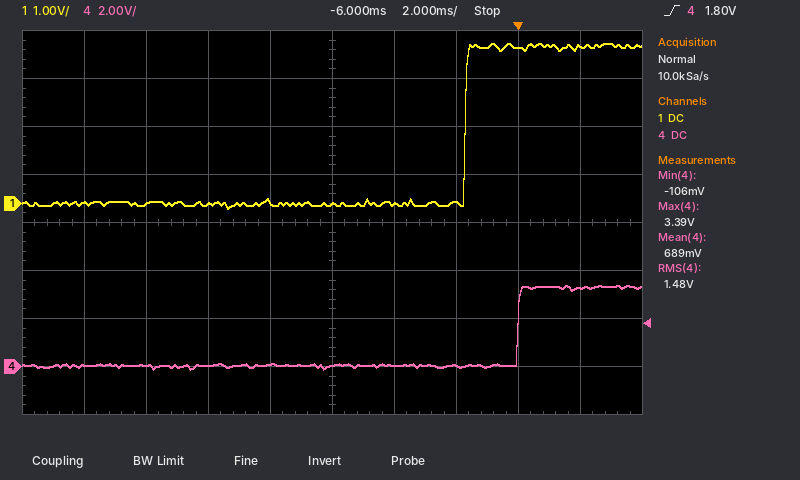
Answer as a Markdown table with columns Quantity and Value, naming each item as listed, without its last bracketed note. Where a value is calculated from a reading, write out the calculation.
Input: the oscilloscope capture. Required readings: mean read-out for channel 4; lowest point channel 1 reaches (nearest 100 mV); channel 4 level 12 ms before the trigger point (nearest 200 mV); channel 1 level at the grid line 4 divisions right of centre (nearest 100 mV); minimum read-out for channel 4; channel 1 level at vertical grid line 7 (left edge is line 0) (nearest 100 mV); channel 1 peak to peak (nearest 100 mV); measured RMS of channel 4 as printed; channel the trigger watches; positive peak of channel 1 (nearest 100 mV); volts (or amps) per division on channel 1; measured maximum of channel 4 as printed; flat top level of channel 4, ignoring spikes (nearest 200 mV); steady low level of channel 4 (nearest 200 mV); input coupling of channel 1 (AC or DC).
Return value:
| Quantity | Value |
|---|---|
| mean read-out for channel 4 | 689 mV |
| lowest point channel 1 reaches | -100 mV |
| channel 4 level 12 ms before the trigger point | 0.0 V |
| channel 1 level at the grid line 4 divisions right of centre | 3.3 V |
| minimum read-out for channel 4 | -106 mV |
| channel 1 level at vertical grid line 7 (left edge is line 0) | 0.0 V |
| channel 1 peak to peak | 3.3 V − (-100 mV) = 3.4 V |
| measured RMS of channel 4 as printed | 1.48 V |
| channel the trigger watches | channel 4 |
| positive peak of channel 1 | 3.3 V |
| volts (or amps) per division on channel 1 | 1 V |
| measured maximum of channel 4 as printed | 3.39 V |
| flat top level of channel 4, ignoring spikes | 3.4 V |
| steady low level of channel 4 | 0.0 V |
| input coupling of channel 1 | DC |
